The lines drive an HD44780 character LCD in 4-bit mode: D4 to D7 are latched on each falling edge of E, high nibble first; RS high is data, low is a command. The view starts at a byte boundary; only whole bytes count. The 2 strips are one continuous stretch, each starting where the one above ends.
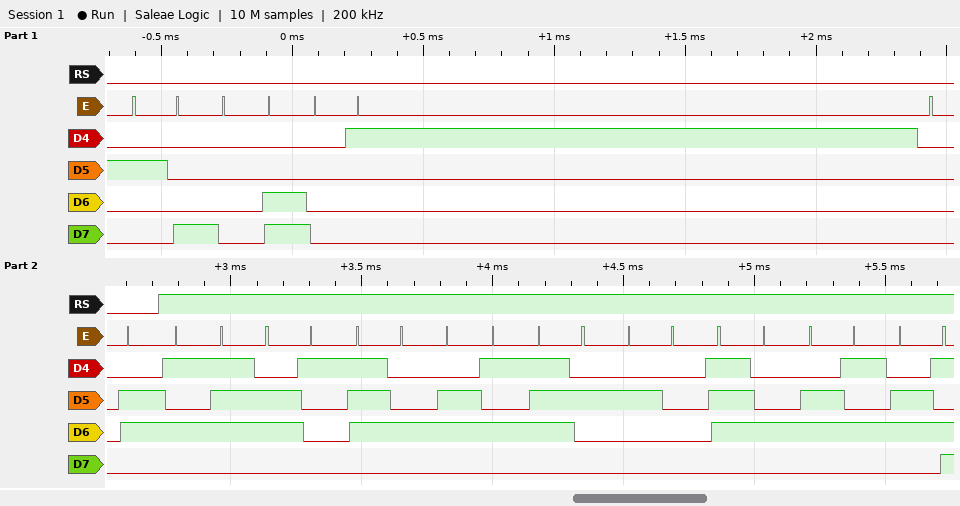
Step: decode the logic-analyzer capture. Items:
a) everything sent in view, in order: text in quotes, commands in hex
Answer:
0x28 0x0C 0x01 0x06 "Water tem"
